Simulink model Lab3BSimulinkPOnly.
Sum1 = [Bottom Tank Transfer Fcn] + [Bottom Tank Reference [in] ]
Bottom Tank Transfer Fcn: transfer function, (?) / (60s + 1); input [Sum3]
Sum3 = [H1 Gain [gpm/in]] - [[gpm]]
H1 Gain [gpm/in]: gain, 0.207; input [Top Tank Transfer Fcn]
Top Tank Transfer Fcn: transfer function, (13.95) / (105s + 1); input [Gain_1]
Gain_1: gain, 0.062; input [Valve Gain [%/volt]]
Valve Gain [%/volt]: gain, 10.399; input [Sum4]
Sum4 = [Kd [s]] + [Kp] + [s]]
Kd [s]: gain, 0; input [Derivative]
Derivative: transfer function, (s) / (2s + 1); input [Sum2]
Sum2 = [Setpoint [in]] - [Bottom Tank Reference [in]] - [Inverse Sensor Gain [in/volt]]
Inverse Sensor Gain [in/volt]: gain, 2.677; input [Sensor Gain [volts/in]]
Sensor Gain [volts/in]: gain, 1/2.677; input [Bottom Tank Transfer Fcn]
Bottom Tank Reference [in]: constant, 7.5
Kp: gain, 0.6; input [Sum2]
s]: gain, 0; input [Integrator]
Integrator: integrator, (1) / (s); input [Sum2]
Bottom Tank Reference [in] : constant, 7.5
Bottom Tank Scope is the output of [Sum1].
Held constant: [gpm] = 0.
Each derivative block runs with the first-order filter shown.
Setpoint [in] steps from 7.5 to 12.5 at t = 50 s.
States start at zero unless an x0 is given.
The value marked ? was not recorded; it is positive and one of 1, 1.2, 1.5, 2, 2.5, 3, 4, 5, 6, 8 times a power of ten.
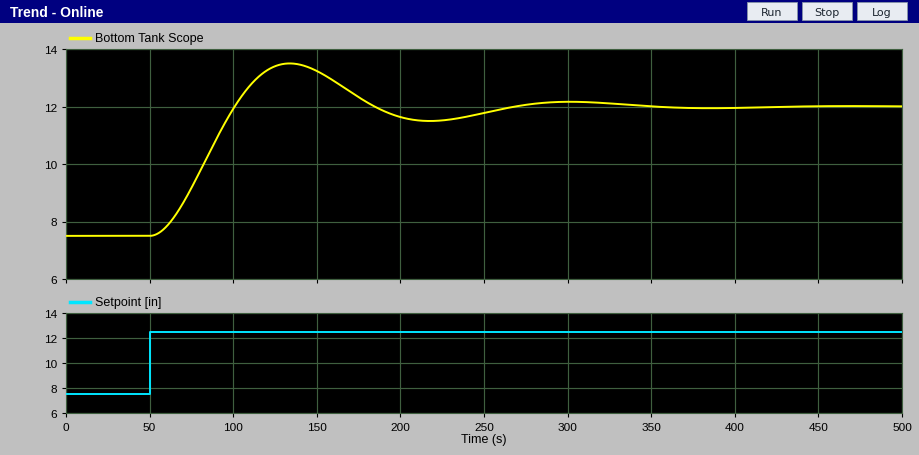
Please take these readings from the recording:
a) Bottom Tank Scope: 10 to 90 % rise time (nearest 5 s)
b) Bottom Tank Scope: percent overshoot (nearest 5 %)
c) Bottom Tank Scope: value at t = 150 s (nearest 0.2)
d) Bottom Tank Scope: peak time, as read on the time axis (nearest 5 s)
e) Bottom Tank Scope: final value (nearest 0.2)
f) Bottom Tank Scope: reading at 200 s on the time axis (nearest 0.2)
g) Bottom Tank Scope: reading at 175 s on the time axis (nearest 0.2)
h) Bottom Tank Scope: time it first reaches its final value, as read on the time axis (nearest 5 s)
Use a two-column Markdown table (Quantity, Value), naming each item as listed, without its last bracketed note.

| Quantity | Value |
|---|---|
| Bottom Tank Scope: 10 to 90 % rise time | 35 s |
| Bottom Tank Scope: percent overshoot | 35 % |
| Bottom Tank Scope: value at t = 150 s | 13.2 |
| Bottom Tank Scope: peak time, as read on the time axis | 135 s |
| Bottom Tank Scope: final value | 12.0 |
| Bottom Tank Scope: reading at 200 s on the time axis | 11.6 |
| Bottom Tank Scope: reading at 175 s on the time axis | 12.4 |
| Bottom Tank Scope: time it first reaches its final value, as read on the time axis | 100 s |
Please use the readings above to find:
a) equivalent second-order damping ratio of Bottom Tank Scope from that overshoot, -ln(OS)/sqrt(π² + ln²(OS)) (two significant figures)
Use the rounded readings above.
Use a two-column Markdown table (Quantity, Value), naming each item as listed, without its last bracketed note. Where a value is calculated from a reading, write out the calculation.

| Quantity | Value |
|---|---|
| equivalent second-order damping ratio of Bottom Tank Scope from that overshoot, -ln(OS)/sqrt(π² + ln²(OS)) | ln(0.35) = -1.050; 1.050 / sqrt(9.870 + 1.102) = 0.32 |
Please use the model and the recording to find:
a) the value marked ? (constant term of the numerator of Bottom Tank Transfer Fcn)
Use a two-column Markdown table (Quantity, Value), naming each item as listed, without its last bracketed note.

| Quantity | Value |
|---|---|
| the value marked ? | 8 |
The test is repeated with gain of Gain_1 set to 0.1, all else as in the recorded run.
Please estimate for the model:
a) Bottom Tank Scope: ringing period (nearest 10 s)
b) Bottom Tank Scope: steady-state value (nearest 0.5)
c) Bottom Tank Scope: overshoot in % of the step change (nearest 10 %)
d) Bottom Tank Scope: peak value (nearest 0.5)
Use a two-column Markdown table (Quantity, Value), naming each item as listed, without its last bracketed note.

| Quantity | Value |
|---|---|
| Bottom Tank Scope: ringing period | 130 s |
| Bottom Tank Scope: steady-state value | 12.0 |
| Bottom Tank Scope: overshoot in % of the step change | 40 % |
| Bottom Tank Scope: peak value | 14.0 |
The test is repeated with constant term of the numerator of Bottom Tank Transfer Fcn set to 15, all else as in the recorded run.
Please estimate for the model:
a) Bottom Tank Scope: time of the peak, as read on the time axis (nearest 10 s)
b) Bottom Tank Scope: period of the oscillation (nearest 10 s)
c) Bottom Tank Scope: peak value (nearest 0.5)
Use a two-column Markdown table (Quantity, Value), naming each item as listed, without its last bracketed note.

| Quantity | Value |
|---|---|
| Bottom Tank Scope: time of the peak, as read on the time axis | 110 s |
| Bottom Tank Scope: period of the oscillation | 120 s |
| Bottom Tank Scope: peak value | 14.5 |
